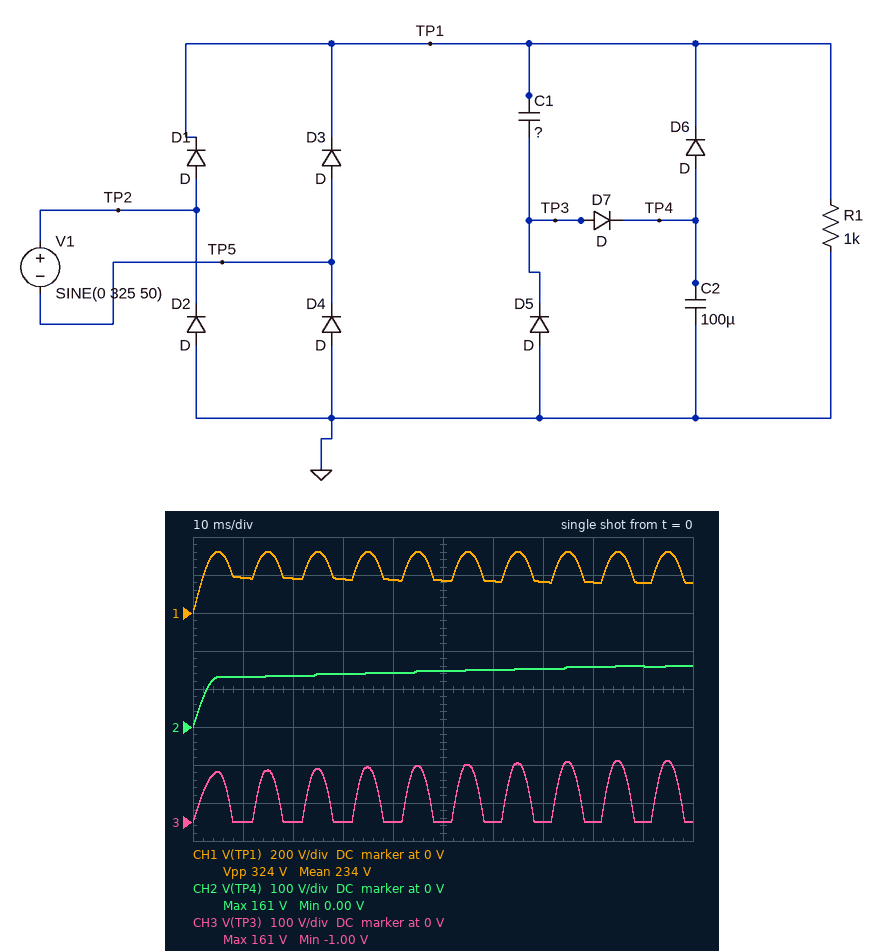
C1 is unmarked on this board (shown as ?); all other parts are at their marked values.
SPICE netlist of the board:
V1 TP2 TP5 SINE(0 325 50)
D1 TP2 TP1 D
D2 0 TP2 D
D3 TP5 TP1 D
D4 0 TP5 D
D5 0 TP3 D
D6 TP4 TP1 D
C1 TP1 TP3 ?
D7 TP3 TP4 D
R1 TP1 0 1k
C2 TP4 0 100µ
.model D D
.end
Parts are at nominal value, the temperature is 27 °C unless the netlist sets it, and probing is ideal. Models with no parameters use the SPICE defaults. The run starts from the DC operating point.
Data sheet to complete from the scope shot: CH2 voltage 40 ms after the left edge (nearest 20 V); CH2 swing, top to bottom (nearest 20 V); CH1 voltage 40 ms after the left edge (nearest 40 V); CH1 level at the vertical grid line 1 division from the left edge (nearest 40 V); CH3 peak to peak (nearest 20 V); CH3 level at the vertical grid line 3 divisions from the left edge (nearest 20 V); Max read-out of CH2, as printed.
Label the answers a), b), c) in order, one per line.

a) 140 V
b) 160 V
c) 160 V
d) 200 V
e) 160 V
f) 0 V
g) 161 V
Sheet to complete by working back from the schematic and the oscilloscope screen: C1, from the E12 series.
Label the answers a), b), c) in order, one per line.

a) 68 µF
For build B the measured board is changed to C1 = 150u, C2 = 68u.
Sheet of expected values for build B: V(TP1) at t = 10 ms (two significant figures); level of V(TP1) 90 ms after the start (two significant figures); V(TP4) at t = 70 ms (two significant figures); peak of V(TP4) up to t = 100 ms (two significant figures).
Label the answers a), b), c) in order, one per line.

a) 210 V
b) 180 V
c) 190 V
d) 220 V
